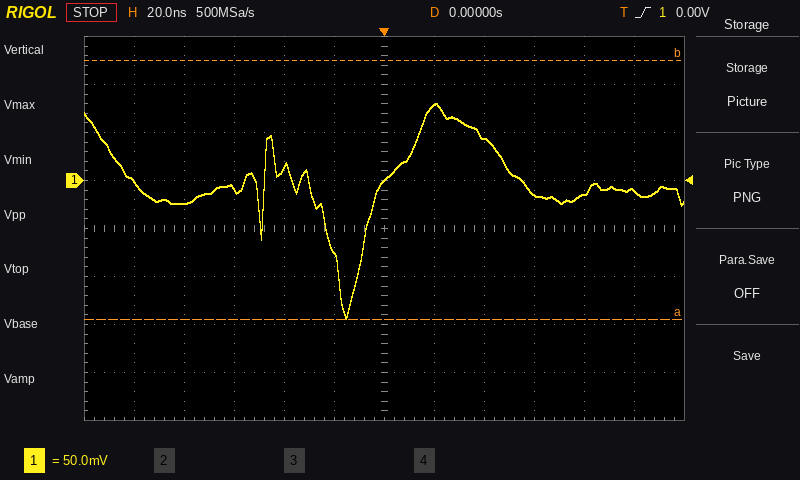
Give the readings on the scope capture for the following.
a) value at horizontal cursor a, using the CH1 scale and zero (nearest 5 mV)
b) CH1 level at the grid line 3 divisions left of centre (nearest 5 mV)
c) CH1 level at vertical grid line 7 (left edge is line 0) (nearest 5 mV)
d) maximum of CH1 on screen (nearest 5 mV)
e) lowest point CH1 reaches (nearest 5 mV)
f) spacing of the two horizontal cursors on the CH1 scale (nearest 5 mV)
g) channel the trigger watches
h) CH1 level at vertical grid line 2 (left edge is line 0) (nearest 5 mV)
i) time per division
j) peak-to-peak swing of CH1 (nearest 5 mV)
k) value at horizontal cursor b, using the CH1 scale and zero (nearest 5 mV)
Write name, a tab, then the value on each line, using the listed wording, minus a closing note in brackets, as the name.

value at horizontal cursor a, using the CH1 scale and zero	-145 mV
CH1 level at the grid line 3 divisions left of centre	-10 mV
CH1 level at vertical grid line 7 (left edge is line 0)	80 mV
maximum of CH1 on screen	80 mV
lowest point CH1 reaches	-145 mV
spacing of the two horizontal cursors on the CH1 scale	270 mV
channel the trigger watches	CH1
CH1 level at vertical grid line 2 (left edge is line 0)	-25 mV
time per division	20 ns
peak-to-peak swing of CH1	225 mV
value at horizontal cursor b, using the CH1 scale and zero	125 mV
